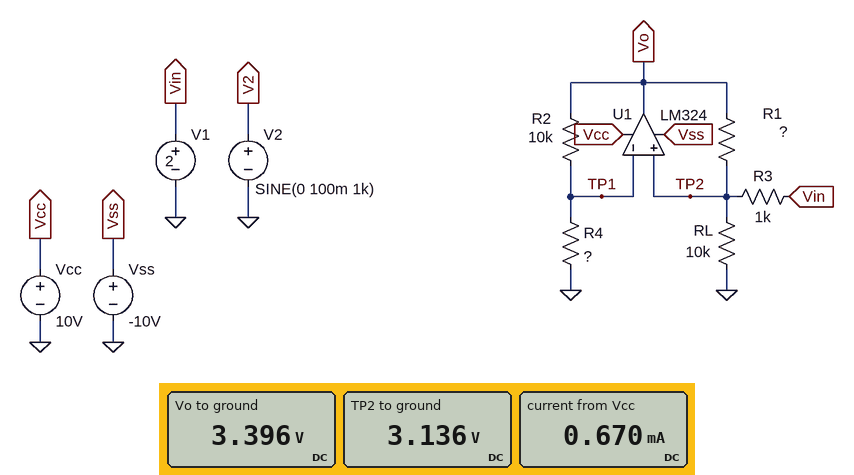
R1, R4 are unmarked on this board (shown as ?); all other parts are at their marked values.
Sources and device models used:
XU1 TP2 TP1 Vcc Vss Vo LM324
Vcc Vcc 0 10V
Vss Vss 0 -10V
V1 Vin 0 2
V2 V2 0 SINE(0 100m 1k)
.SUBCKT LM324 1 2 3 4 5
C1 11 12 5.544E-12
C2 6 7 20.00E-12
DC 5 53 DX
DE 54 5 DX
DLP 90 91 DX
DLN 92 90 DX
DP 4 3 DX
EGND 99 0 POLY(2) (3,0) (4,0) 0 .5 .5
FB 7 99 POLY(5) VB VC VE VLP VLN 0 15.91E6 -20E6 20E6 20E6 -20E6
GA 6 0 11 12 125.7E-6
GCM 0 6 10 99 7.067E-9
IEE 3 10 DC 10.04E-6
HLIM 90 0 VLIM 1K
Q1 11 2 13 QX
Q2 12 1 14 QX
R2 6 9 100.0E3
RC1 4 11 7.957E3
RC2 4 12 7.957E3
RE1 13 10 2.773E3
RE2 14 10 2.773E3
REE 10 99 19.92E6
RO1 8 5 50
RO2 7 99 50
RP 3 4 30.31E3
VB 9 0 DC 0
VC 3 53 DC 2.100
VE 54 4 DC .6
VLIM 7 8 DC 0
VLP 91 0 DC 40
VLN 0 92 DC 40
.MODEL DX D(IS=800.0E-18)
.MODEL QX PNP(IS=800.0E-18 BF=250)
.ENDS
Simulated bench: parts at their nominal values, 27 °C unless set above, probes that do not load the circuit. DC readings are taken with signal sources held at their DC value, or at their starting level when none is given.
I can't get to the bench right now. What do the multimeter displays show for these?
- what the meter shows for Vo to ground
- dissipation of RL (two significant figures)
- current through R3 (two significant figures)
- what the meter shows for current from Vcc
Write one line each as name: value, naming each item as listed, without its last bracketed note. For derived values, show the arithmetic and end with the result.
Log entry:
what the meter shows for Vo to ground: 3.396 V
dissipation of RL: (3.136 V)^2 / 10 kΩ = 980 µW
current through R3: (3.136 V - 2 V) / 1 kΩ = 1.1 mA
what the meter shows for current from Vcc: 0.670 mA
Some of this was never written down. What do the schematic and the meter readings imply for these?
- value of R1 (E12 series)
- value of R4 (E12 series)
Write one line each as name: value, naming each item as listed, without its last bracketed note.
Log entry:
value of R1: 180 Ω
value of R4: 120 kΩ
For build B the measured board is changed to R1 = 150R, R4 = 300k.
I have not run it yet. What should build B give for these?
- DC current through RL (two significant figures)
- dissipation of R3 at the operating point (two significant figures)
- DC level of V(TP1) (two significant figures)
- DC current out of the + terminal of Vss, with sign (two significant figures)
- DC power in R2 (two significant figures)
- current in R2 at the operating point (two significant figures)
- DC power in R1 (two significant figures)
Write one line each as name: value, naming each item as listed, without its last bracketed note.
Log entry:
DC current through RL: 230 µA
dissipation of R3 at the operating point: 76 µW
DC level of V(TP1): 2.3 V
DC current out of the + terminal of Vss, with sign: -670 µA
DC power in R2: 570 nW
current in R2 at the operating point: 7.6 µA
DC power in R1: 38 µW
